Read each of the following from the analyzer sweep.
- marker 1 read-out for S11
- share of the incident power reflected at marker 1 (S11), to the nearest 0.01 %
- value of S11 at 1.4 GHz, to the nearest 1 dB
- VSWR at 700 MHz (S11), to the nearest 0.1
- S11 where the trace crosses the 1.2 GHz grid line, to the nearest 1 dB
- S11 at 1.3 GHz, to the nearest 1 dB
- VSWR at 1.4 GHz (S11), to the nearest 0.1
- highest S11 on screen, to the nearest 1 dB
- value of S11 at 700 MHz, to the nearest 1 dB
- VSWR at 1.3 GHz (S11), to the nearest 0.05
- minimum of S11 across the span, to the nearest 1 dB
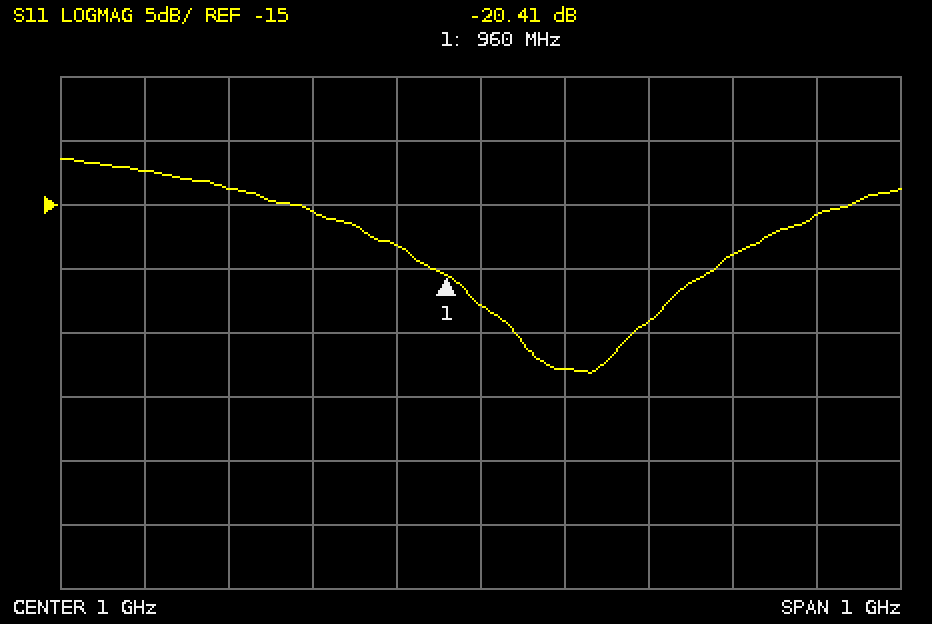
-20.41 dB
0.91 %
-16 dB
1.5
-24 dB
-19 dB
1.4
-11 dB
-14 dB
1.25
-28 dB
